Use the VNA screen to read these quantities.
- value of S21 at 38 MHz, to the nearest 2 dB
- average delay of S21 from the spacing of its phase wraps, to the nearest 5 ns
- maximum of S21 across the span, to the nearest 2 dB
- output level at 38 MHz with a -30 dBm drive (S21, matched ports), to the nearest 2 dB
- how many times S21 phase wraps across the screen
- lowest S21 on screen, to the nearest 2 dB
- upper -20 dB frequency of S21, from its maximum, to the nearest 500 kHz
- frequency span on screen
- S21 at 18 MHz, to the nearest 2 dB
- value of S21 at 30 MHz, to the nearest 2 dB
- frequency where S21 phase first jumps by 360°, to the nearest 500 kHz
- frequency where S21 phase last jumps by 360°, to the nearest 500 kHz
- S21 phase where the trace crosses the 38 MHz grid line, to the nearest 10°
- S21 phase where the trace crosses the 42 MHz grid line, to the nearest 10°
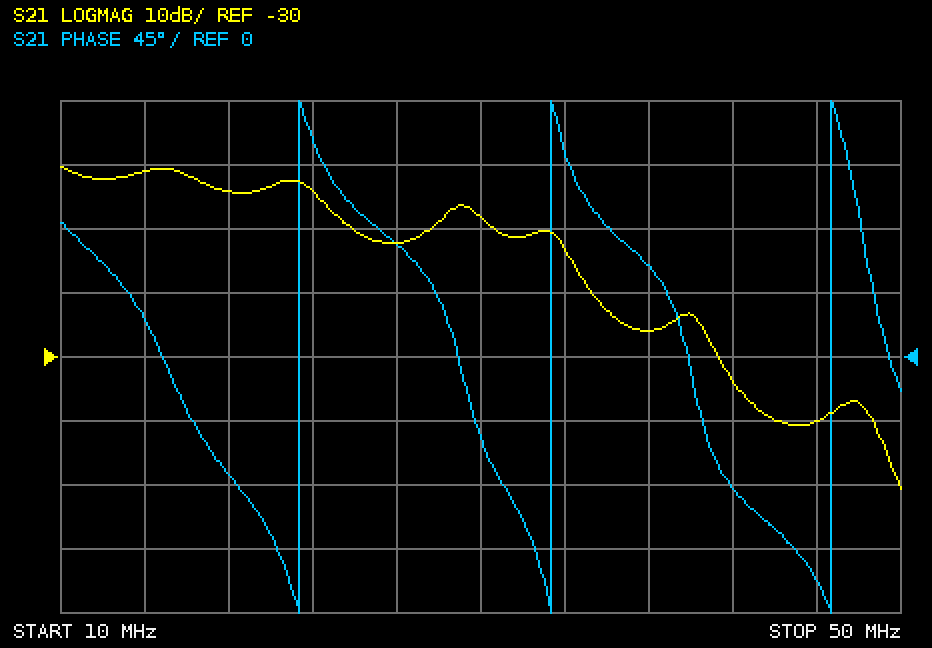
-26 dB
80 ns
0 dB
-56 dBm
3
-50 dB
35.5 MHz
40 MHz
-4 dB
-8 dB
21.5 MHz
46.5 MHz
60°
-90°
